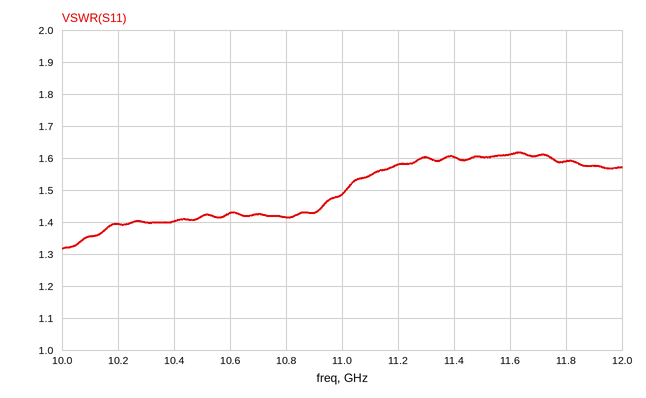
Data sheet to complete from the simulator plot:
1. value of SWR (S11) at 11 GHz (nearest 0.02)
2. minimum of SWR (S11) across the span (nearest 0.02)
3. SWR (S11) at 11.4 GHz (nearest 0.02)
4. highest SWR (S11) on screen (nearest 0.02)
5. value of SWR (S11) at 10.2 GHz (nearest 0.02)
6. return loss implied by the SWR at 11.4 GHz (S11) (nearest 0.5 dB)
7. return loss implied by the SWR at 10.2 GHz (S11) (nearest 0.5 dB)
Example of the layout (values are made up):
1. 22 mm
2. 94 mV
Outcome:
1. 1.48
2. 1.32
3. 1.60
4. 1.62
5. 1.40
6. 12.5 dB
7. 15.5 dB
